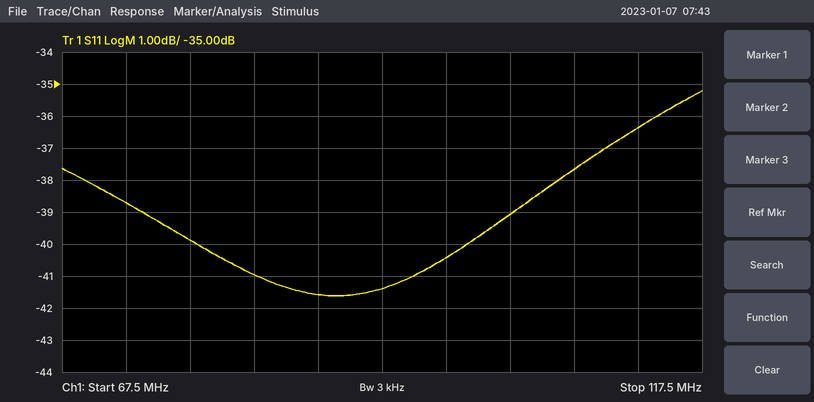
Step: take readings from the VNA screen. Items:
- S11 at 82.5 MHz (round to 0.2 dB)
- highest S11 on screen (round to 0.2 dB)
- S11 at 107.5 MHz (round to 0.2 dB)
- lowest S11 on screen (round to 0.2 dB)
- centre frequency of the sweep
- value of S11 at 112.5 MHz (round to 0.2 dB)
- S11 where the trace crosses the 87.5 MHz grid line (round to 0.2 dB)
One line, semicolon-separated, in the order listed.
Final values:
-41.0 dB; -35.2 dB; -37.6 dB; -41.6 dB; 92.5 MHz; -36.4 dB; -41.6 dB
